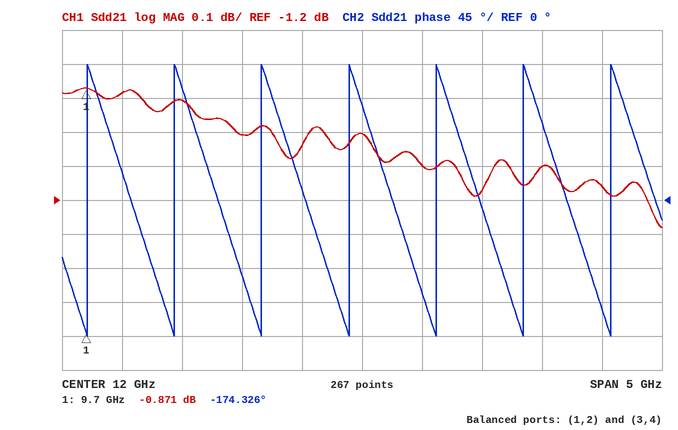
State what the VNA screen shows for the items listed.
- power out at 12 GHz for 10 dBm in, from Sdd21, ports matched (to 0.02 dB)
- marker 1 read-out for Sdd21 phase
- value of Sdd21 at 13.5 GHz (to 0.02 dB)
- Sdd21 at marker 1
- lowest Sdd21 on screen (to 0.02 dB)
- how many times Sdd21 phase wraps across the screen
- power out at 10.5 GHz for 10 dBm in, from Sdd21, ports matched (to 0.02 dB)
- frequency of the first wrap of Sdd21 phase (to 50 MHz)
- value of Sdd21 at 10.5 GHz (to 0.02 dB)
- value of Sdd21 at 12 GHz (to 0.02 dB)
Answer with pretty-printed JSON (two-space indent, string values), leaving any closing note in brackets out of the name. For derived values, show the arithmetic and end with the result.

{
  "power out at 12 GHz for 10 dBm in, from Sdd21, ports matched": "10 dBm + (-1.00 dB) = 9.00 dBm",
  "marker 1 read-out for Sdd21 phase": "-174.326°",
  "value of Sdd21 at 13.5 GHz": "-1.10 dB",
  "Sdd21 at marker 1": "-0.871 dB",
  "lowest Sdd21 on screen": "-1.28 dB",
  "how many times Sdd21 phase wraps across the screen": "7",
  "power out at 10.5 GHz for 10 dBm in, from Sdd21, ports matched": "10 dBm + (-0.90 dB) = 9.10 dBm",
  "frequency of the first wrap of Sdd21 phase": "9.70 GHz",
  "value of Sdd21 at 10.5 GHz": "-0.90 dB",
  "value of Sdd21 at 12 GHz": "-1.00 dB"
}
